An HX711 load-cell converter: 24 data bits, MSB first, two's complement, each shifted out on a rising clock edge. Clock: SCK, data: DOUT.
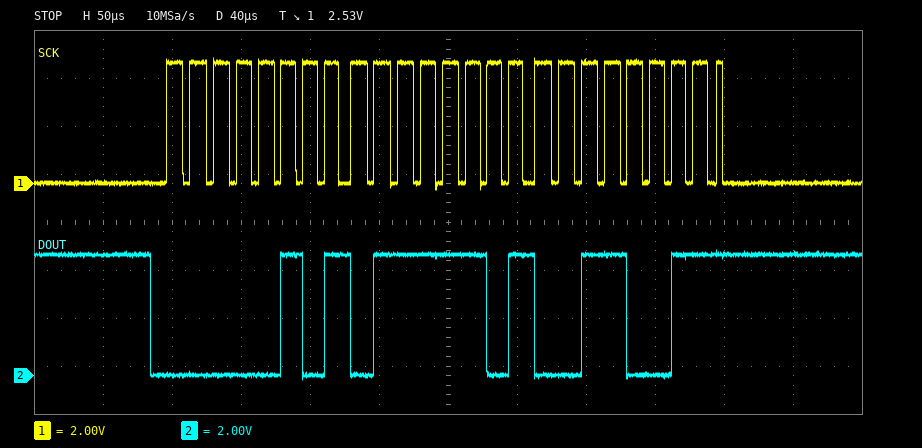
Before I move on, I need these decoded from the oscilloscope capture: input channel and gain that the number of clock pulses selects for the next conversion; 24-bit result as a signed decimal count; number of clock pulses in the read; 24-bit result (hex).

channel A, gain 128
359731
25
0x057D33
